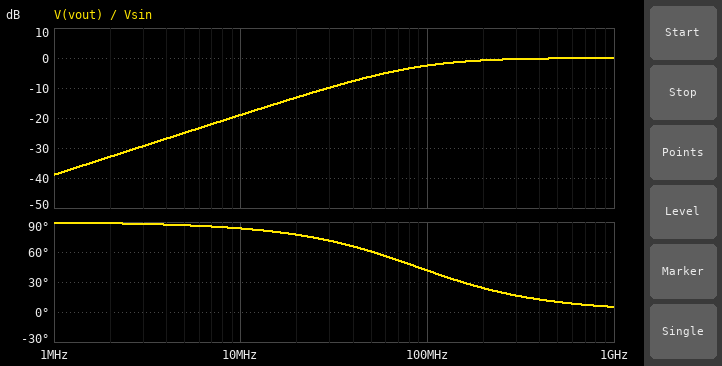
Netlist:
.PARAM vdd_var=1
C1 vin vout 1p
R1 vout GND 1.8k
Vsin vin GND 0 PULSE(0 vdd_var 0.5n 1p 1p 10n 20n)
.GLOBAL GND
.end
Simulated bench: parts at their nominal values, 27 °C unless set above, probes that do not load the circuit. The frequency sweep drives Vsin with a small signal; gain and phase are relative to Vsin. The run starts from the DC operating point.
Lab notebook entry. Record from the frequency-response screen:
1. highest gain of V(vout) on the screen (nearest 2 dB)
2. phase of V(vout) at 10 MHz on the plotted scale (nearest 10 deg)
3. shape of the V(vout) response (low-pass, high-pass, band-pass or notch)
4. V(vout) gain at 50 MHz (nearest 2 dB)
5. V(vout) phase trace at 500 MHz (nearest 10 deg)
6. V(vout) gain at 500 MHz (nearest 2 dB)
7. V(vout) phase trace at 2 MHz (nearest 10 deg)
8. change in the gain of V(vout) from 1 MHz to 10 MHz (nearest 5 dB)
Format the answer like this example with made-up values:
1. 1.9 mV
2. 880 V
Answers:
1. 0 dB
2. 80 deg
3. high-pass
4. -6 dB
5. 10 deg
6. 0 dB
7. 90 deg
8. 20 dB
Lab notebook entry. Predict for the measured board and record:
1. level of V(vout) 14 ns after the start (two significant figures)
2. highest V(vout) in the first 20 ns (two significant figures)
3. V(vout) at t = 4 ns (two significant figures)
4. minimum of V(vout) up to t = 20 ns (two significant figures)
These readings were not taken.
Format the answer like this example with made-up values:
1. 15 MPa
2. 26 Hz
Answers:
1. -140 mV
2. 1.0 V
3. 140 mV
4. -1.0 V
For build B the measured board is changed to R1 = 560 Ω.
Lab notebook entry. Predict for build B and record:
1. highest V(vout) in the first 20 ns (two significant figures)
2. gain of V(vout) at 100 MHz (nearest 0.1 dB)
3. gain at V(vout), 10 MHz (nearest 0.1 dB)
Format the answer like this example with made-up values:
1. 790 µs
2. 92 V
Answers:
1. 1.0 V
2. -9.6 dB
3. -29.1 dB
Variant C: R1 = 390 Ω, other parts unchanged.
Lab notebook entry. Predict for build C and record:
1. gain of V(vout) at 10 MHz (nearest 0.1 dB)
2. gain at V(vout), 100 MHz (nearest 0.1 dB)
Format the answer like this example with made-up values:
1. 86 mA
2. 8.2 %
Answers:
1. -32.2 dB
2. -12.5 dB
